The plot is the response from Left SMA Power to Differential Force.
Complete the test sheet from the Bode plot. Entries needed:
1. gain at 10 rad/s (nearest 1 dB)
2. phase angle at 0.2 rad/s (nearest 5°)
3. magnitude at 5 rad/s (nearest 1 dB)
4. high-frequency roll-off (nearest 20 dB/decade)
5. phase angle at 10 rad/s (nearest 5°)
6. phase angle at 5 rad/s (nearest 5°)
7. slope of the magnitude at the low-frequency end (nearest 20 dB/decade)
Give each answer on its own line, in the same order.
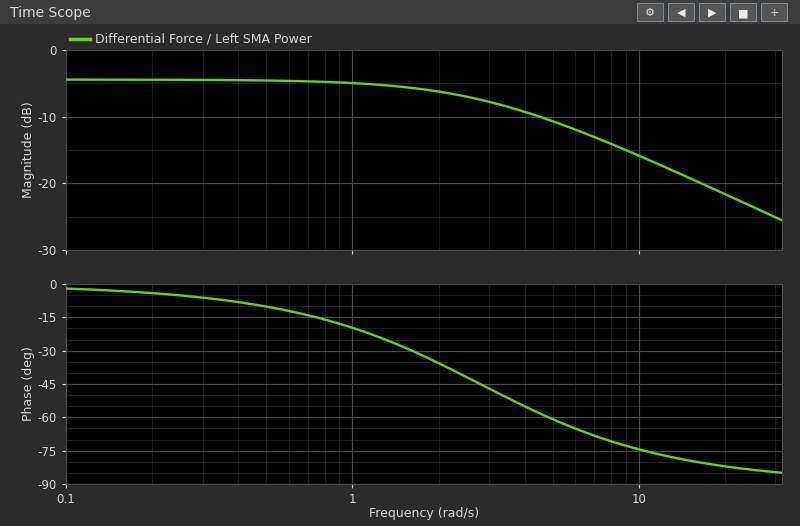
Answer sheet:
-16 dB
-5°
-11 dB
-20 dB/decade
-75°
-60°
0 dB/decade
